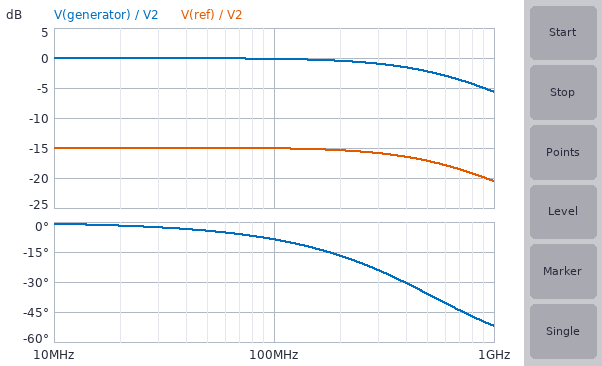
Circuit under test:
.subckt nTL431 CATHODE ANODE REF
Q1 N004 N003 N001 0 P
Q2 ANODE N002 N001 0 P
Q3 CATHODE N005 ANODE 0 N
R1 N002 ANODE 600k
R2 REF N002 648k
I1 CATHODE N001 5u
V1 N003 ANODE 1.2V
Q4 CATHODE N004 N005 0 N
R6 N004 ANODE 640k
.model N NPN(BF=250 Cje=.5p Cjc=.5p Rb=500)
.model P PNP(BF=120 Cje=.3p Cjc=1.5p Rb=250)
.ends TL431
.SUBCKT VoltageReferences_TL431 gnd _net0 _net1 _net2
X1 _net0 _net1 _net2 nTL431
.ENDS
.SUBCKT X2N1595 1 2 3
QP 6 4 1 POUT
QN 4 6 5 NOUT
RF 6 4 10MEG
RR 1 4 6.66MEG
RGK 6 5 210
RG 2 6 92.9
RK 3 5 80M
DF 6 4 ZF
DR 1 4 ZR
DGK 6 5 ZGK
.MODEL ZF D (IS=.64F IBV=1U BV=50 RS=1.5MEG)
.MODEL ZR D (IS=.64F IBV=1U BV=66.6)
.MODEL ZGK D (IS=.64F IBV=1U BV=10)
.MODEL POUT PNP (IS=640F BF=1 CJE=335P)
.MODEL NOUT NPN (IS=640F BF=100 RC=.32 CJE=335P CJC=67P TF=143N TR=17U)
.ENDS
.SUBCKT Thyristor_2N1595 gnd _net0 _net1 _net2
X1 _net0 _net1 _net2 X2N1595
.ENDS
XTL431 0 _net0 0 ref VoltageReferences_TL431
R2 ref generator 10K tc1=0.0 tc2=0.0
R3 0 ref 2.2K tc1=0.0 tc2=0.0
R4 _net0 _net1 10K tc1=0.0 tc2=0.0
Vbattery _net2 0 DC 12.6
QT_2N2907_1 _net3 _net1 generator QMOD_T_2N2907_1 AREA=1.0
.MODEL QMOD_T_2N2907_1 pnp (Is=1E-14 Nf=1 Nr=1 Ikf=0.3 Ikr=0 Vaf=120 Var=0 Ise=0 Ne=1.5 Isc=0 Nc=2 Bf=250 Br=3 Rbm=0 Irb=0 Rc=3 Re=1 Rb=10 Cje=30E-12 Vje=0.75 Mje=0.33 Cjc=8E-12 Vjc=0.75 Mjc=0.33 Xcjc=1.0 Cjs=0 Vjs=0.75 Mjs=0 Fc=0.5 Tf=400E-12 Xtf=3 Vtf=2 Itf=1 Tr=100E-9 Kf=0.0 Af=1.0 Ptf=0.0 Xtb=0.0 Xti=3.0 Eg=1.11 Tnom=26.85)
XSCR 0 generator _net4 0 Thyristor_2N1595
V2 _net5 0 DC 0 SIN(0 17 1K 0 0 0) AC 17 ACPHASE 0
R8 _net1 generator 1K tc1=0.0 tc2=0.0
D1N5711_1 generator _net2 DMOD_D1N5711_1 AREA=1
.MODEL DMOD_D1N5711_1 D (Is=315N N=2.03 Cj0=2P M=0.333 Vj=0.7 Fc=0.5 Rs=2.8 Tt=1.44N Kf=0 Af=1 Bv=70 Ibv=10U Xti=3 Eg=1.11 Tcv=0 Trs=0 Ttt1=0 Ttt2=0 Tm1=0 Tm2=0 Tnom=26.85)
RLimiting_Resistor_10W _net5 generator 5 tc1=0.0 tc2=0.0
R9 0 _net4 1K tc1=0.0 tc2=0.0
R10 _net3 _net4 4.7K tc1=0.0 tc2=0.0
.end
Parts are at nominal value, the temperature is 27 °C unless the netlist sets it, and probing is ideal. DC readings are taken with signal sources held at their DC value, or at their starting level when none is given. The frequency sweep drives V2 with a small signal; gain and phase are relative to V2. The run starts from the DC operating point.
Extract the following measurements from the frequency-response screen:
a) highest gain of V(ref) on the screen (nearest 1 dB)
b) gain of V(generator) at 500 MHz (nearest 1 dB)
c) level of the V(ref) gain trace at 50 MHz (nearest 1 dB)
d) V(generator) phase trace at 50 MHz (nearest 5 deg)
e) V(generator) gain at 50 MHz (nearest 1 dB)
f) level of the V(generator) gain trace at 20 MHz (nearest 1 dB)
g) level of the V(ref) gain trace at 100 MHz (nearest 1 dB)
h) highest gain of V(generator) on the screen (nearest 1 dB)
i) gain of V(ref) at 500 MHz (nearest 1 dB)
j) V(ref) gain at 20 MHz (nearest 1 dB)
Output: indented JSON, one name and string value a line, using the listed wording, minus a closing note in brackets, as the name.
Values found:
{
  "highest gain of V(ref) on the screen": "-15 dB",
  "gain of V(generator) at 500 MHz": "-2 dB",
  "level of the V(ref) gain trace at 50 MHz": "-15 dB",
  "V(generator) phase trace at 50 MHz": "-5 deg",
  "V(generator) gain at 50 MHz": "0 dB",
  "level of the V(generator) gain trace at 20 MHz": "0 dB",
  "level of the V(ref) gain trace at 100 MHz": "-15 dB",
  "highest gain of V(generator) on the screen": "0 dB",
  "gain of V(ref) at 500 MHz": "-17 dB",
  "V(ref) gain at 20 MHz": "-15 dB"
}
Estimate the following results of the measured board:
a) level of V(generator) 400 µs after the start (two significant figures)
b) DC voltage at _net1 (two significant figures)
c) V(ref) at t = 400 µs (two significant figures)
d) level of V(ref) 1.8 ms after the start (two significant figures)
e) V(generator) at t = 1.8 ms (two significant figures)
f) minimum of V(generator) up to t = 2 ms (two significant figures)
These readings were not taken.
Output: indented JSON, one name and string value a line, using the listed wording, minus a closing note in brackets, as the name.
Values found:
{
  "level of V(generator) 400 µs after the start": "1.2 V",
  "DC voltage at _net1": "-5.0 mV",
  "V(ref) at t = 400 µs": "210 mV",
  "level of V(ref) 1.8 ms after the start": "-2.9 V",
  "V(generator) at t = 1.8 ms": "-16 V",
  "minimum of V(generator) up to t = 2 ms": "-17 V"
}
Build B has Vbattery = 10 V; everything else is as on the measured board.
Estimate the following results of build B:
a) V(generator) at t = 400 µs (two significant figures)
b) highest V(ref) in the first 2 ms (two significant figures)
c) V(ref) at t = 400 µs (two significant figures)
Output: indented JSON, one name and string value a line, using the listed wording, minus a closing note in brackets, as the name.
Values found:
{
  "V(generator) at t = 400 µs": "10 V",
  "highest V(ref) in the first 2 ms": "2.3 V",
  "V(ref) at t = 400 µs": "1.8 V"
}
